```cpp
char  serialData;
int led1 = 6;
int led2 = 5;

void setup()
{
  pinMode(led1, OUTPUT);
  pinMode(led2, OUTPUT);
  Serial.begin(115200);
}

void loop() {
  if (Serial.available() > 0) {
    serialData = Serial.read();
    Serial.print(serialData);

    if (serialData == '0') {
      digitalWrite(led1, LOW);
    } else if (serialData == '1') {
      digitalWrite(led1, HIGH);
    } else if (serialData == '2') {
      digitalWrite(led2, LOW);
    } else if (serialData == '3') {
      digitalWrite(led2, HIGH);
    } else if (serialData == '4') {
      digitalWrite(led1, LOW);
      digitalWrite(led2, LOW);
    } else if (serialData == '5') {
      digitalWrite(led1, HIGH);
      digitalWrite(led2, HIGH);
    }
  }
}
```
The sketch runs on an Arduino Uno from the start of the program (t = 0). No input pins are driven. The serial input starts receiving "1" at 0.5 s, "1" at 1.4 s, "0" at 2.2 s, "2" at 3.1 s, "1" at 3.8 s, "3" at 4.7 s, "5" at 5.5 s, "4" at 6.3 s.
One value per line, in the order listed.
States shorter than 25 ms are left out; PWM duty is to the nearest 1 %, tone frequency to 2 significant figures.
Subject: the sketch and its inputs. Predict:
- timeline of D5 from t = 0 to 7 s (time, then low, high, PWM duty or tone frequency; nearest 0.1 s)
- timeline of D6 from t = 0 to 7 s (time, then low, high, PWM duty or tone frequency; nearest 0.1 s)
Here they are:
0 s low; 4.7 s high; 6.3 s low
0 s low; 0.5 s high; 2.2 s low; 3.8 s high; 6.3 s low
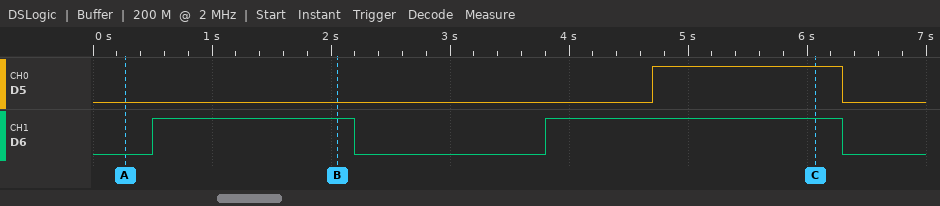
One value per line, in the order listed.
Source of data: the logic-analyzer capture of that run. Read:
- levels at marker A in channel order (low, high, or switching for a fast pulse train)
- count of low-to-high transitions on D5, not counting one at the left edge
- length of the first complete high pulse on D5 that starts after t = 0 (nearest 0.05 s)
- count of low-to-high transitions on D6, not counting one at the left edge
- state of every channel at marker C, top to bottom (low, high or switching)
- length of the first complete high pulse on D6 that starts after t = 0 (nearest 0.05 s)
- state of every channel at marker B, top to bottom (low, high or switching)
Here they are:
D5 low, D6 low
1
1.60 s
2
D5 high, D6 high
1.70 s
D5 low, D6 high
